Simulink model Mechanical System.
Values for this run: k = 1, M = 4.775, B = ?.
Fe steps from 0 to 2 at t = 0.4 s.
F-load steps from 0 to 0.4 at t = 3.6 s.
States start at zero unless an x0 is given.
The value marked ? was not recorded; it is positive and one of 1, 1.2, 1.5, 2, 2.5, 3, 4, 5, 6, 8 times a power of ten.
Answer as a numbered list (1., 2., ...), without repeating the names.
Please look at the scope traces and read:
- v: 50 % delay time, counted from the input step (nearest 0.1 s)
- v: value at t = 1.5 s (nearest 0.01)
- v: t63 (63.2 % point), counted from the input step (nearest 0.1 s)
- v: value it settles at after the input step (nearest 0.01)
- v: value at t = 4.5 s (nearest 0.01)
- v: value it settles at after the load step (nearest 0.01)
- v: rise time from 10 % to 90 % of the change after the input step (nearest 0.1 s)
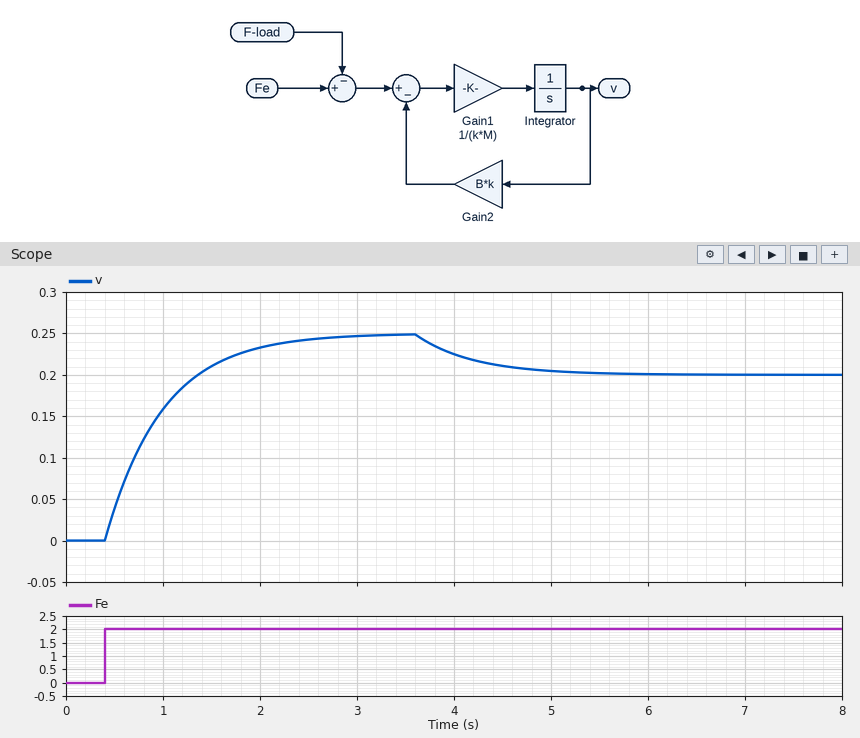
1. 0.4 s
2. 0.21
3. 0.6 s
4. 0.25
5. 0.21
6. 0.20
7. 1.3 s
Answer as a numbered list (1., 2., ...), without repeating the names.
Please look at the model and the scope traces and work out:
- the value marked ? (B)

1. 8
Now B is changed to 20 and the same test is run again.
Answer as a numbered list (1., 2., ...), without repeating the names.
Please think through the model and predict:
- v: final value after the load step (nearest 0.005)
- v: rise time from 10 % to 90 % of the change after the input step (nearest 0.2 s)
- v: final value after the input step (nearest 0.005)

1. 0.080
2. 0.6 s
3. 0.100
